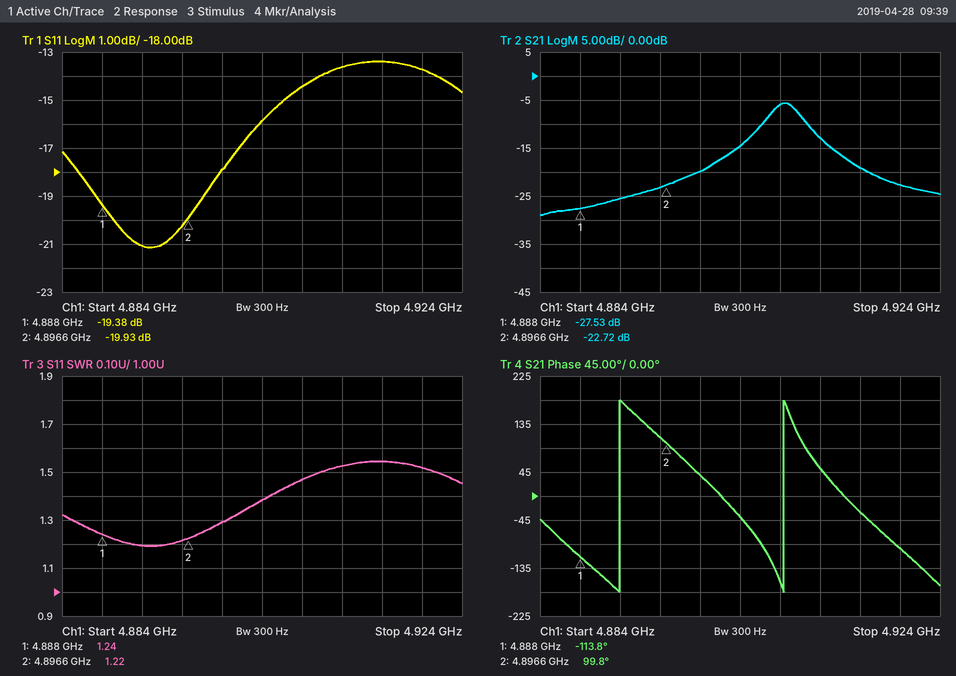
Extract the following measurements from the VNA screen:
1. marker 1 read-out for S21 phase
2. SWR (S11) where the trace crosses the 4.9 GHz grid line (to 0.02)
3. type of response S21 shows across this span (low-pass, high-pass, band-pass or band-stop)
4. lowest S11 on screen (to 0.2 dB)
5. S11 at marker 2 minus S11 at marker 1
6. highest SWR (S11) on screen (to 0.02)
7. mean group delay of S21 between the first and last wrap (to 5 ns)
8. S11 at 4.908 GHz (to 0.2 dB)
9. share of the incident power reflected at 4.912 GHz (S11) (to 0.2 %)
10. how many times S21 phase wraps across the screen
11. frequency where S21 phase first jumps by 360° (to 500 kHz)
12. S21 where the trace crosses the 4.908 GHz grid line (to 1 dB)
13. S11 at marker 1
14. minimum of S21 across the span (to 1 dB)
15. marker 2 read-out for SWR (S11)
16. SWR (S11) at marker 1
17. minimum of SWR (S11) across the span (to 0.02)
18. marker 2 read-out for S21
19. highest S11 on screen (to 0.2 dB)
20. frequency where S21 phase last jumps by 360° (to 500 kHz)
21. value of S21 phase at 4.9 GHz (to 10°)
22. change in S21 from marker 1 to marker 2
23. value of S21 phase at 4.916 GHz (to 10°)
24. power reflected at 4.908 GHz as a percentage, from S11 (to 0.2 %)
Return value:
-113.8°
1.30
band-pass
-21.2 dB
-0.55 dB
1.54
60 ns
-14.4 dB
4.4 %
2
4.8920 GHz
-6 dB
-19.38 dB
-29 dB
1.22
1.24
1.20
-22.72 dB
-13.4 dB
4.9085 GHz
40°
4.81 dB
-30°
3.6 %
